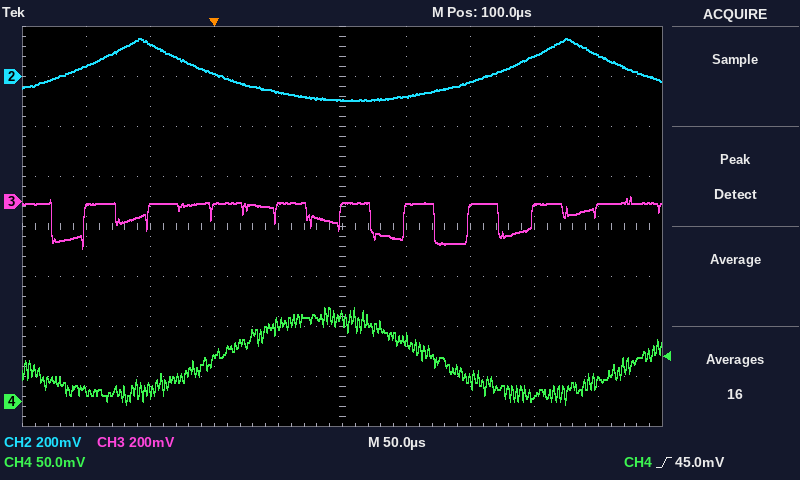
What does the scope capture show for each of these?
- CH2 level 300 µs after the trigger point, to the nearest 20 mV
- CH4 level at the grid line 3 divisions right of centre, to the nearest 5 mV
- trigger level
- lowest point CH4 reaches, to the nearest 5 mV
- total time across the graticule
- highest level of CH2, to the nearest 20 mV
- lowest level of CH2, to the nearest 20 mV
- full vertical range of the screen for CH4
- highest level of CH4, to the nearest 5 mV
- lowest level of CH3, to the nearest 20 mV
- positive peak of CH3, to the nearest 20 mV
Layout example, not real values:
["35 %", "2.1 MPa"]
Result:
["80 mV", "5 mV", "45.0 mV", "-5 mV", "500 µs", "160 mV", "-100 mV", "400 mV", "95 mV", "-180 mV", "20 mV"]
